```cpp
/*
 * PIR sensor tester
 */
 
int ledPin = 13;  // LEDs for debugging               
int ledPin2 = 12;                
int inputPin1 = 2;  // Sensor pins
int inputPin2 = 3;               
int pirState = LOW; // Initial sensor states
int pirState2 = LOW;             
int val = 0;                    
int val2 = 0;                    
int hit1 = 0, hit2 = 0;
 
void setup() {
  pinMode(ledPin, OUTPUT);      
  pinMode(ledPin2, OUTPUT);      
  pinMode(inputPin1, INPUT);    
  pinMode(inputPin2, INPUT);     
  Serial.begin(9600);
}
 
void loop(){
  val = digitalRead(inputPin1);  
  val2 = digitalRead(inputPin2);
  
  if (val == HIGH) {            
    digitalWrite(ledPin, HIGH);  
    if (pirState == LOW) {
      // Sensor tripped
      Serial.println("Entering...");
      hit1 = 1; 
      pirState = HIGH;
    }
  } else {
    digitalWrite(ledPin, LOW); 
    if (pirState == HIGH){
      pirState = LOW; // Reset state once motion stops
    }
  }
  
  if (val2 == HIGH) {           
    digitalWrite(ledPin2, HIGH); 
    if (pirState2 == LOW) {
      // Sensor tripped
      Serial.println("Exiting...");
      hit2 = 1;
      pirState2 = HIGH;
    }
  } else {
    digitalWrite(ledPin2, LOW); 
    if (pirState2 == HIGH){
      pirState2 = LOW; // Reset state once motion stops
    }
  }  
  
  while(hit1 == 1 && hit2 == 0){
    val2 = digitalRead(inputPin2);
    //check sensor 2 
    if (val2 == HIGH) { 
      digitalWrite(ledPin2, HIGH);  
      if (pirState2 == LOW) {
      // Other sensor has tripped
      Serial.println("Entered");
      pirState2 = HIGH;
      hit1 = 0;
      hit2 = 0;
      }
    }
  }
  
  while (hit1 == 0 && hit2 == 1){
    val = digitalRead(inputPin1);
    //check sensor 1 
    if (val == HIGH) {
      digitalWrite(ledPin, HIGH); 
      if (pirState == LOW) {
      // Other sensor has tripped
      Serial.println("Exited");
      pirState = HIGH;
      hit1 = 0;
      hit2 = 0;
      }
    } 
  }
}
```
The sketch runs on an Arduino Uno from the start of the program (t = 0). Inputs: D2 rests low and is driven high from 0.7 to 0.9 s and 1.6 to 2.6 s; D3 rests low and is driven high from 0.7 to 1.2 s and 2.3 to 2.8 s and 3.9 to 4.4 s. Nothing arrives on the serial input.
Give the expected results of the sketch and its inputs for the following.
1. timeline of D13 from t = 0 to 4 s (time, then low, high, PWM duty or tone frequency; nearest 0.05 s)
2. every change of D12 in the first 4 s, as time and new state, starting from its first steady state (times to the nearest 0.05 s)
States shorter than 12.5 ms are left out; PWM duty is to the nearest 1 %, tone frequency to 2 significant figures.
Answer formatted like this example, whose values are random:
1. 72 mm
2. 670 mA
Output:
1. 0 s low; 0.7 s high; 0.9 s low; 1.6 s high; 2.6 s low
2. 0 s low; 0.7 s high; 1.2 s low; 2.3 s high; 2.8 s low; 3.9 s high
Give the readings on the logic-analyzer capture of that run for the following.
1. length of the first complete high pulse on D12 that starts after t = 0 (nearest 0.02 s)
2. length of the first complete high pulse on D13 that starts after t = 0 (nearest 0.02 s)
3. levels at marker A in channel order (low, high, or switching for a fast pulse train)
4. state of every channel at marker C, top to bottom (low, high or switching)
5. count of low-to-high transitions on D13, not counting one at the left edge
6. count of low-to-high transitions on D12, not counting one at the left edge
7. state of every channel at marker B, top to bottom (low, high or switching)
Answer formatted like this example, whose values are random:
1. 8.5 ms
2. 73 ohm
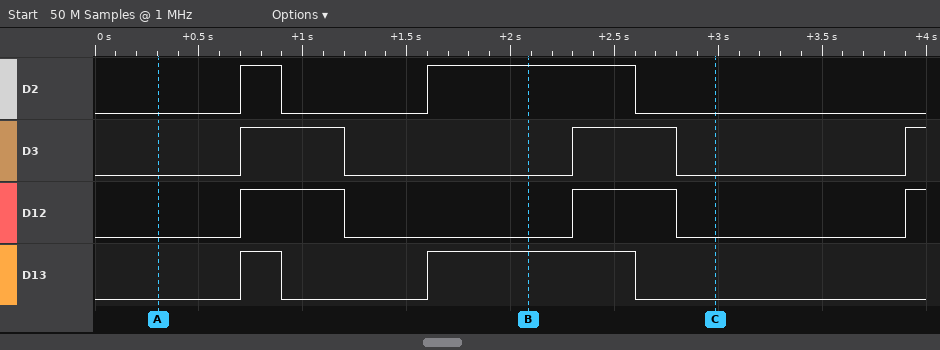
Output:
1. 0.50 s
2. 0.20 s
3. D2 low, D3 low, D12 low, D13 low
4. D2 low, D3 low, D12 low, D13 low
5. 2
6. 3
7. D2 high, D3 low, D12 low, D13 high
